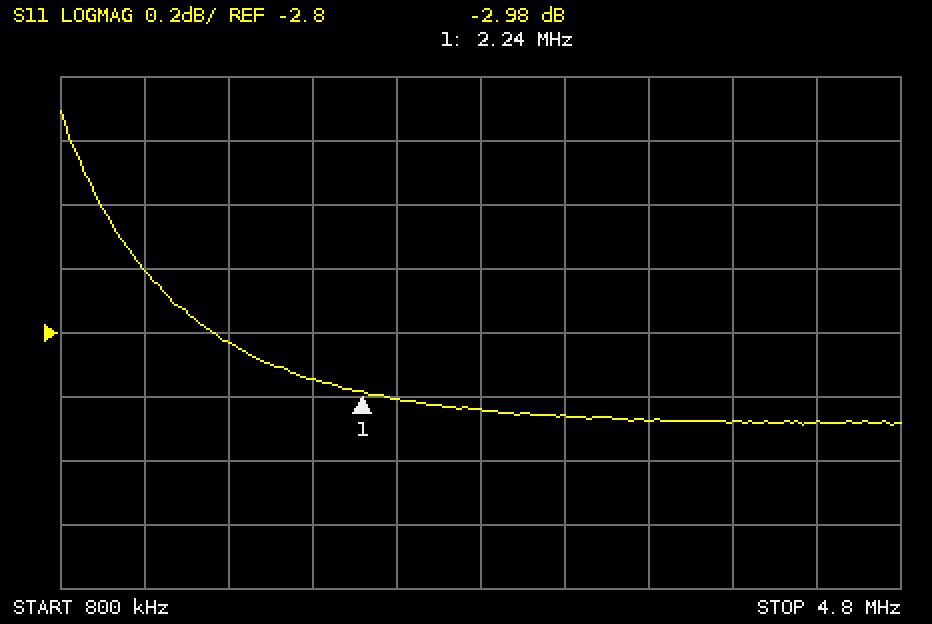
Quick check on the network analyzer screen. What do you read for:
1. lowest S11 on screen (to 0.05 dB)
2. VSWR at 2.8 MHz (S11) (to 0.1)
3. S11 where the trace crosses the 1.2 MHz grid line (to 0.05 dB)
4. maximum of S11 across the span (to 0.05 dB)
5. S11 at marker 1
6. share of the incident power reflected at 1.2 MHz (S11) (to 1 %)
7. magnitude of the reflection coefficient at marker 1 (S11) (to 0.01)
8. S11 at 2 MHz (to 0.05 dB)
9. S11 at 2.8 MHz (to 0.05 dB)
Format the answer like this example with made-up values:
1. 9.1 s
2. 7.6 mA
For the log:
1. -3.10 dB
2. 5.8
3. -2.60 dB
4. -2.10 dB
5. -2.98 dB
6. 55 %
7. 0.71
8. -2.95 dB
9. -3.05 dB
